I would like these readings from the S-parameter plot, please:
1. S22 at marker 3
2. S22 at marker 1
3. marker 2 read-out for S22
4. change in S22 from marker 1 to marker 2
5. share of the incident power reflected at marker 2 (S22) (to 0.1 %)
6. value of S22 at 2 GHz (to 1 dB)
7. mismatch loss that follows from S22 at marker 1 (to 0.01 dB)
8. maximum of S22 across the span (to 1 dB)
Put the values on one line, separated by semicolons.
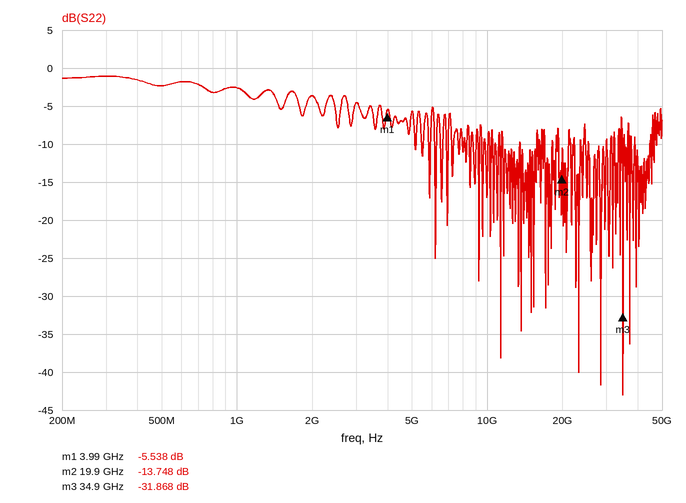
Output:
-31.868 dB; -5.538 dB; -13.748 dB; -8.210 dB; 4.2 %; -4 dB; 1.42 dB; -1 dB
